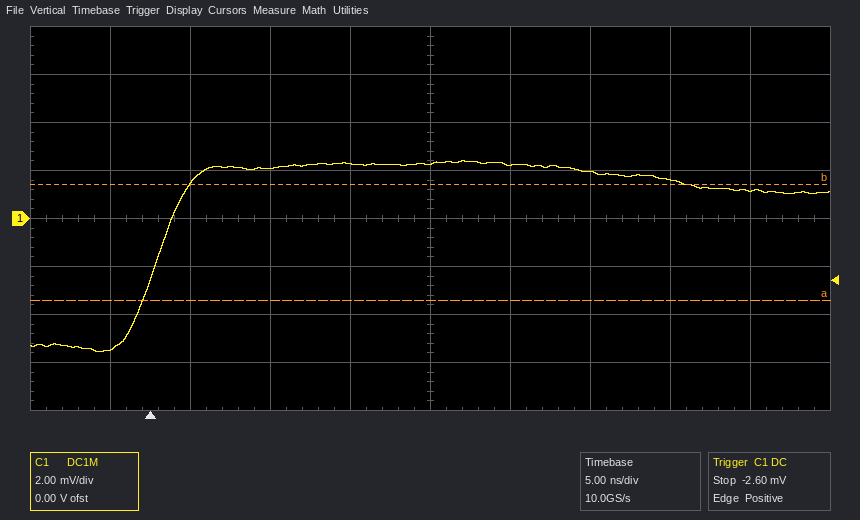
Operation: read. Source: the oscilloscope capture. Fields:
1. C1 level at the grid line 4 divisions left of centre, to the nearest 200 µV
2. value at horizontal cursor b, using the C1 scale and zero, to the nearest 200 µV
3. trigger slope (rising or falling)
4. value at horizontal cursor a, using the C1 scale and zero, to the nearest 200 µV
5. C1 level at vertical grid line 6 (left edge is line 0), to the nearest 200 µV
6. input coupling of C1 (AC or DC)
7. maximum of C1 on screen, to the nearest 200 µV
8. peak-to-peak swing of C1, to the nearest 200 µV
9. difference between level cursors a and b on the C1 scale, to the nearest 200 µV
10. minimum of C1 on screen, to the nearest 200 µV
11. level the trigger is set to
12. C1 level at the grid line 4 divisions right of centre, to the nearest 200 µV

-5.4 mV
1.4 mV
rising
-3.4 mV
2.2 mV
DC
2.4 mV
8.0 mV
4.8 mV
-5.6 mV
-2.60 mV
1.2 mV
